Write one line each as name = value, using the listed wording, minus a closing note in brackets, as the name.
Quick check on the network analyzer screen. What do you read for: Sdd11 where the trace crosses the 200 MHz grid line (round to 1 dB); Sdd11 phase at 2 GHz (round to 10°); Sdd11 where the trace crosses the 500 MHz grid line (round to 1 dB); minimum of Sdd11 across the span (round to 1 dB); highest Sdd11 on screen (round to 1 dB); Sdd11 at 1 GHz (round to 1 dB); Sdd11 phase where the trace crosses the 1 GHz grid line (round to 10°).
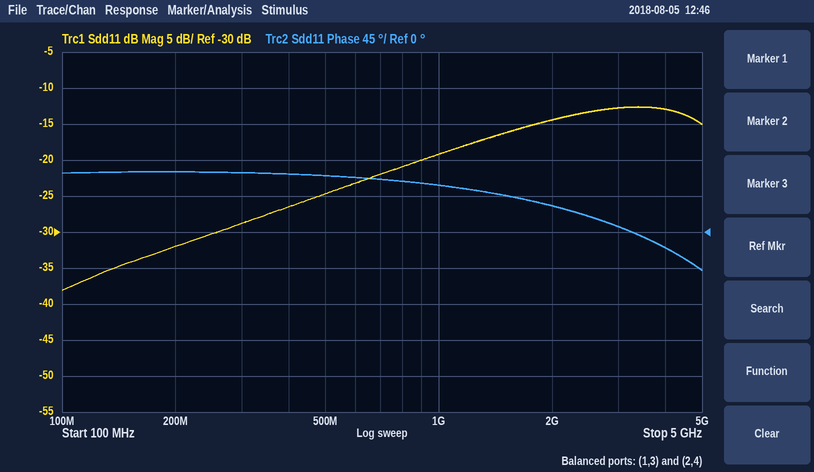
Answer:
Sdd11 where the trace crosses the 200 MHz grid line = -32 dB
Sdd11 phase at 2 GHz = 30°
Sdd11 where the trace crosses the 500 MHz grid line = -25 dB
minimum of Sdd11 across the span = -38 dB
highest Sdd11 on screen = -13 dB
Sdd11 at 1 GHz = -19 dB
Sdd11 phase where the trace crosses the 1 GHz grid line = 60°
